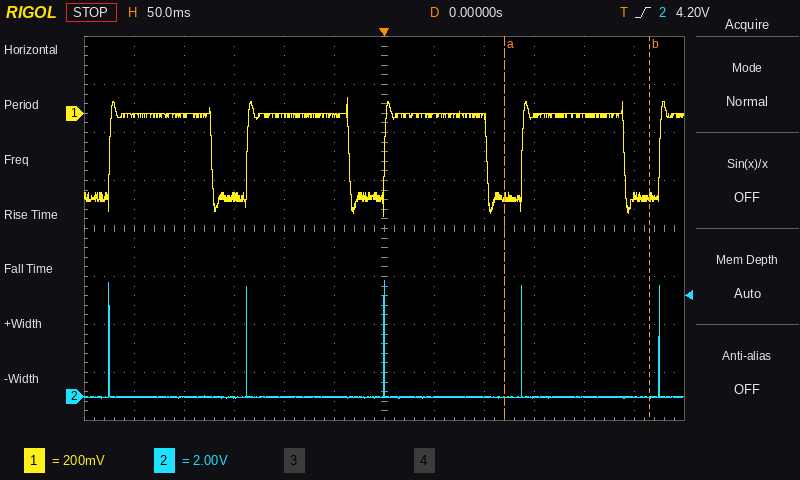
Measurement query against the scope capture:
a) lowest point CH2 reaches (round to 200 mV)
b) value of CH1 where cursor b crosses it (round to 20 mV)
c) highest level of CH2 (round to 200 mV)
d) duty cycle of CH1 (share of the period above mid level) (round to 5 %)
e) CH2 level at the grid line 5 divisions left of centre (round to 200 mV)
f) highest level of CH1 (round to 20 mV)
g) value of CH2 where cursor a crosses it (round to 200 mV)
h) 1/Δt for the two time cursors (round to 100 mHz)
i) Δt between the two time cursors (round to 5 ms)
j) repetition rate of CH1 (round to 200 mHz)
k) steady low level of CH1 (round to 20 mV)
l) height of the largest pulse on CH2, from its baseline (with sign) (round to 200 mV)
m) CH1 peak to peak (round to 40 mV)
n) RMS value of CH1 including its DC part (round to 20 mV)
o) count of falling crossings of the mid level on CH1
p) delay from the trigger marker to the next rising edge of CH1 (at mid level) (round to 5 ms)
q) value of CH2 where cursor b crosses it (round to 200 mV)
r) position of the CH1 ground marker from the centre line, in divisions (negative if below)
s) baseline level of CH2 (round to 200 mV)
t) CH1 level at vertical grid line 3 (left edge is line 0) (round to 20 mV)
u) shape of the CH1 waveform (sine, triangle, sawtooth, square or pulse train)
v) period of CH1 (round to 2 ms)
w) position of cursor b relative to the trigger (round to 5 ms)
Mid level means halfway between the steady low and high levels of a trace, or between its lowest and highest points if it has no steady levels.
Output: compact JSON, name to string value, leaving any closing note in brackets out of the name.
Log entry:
{"lowest point CH2 reaches": "0.0 V", "value of CH1 where cursor b crosses it": "-340 mV", "highest level of CH2": "4.8 V", "duty cycle of CH1 (share of the period above mid level)": "75 %", "CH2 level at the grid line 5 divisions left of centre": "0.0 V", "highest level of CH1": "60 mV", "value of CH2 where cursor a crosses it": "0.0 V", "1/Δt for the two time cursors": "6.9 Hz", "Δt between the two time cursors": "145 ms", "repetition rate of CH1": "7.2 Hz", "steady low level of CH1": "-360 mV", "height of the largest pulse on CH2, from its baseline (with sign)": "+4.8 V", "CH1 peak to peak": "480 mV", "RMS value of CH1 including its DC part": "180 mV", "count of falling crossings of the mid level on CH1": "4", "delay from the trigger marker to the next rising edge of CH1 (at mid level)": "140 ms", "value of CH2 where cursor b crosses it": "0.0 V", "position of the CH1 ground marker from the centre line, in divisions": "+2.4 div", "baseline level of CH2": "0.0 V", "CH1 level at vertical grid line 3 (left edge is line 0)": "-340 mV", "shape of the CH1 waveform": "pulse train", "period of CH1": "138 ms", "position of cursor b relative to the trigger": "+265 ms"}
